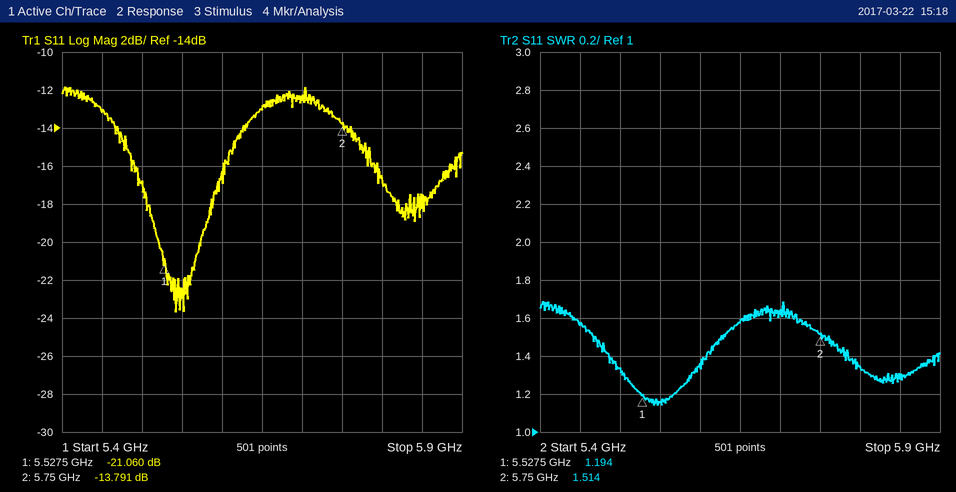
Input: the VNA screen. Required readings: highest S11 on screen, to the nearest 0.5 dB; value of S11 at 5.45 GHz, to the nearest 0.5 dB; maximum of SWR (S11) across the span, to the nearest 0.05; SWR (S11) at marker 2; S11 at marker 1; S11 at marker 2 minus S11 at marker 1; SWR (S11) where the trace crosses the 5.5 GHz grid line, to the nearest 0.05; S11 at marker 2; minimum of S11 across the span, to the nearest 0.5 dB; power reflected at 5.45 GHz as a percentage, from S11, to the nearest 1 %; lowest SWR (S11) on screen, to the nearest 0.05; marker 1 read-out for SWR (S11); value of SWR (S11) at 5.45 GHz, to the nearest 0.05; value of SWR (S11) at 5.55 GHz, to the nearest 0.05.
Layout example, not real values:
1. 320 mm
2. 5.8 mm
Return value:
1. -12.0 dB
2. -13.0 dB
3. 1.70
4. 1.514
5. -21.060 dB
6. 7.269 dB
7. 1.35
8. -13.791 dB
9. -23.5 dB
10. 5 %
11. 1.15
12. 1.194
13. 1.55
14. 1.15
